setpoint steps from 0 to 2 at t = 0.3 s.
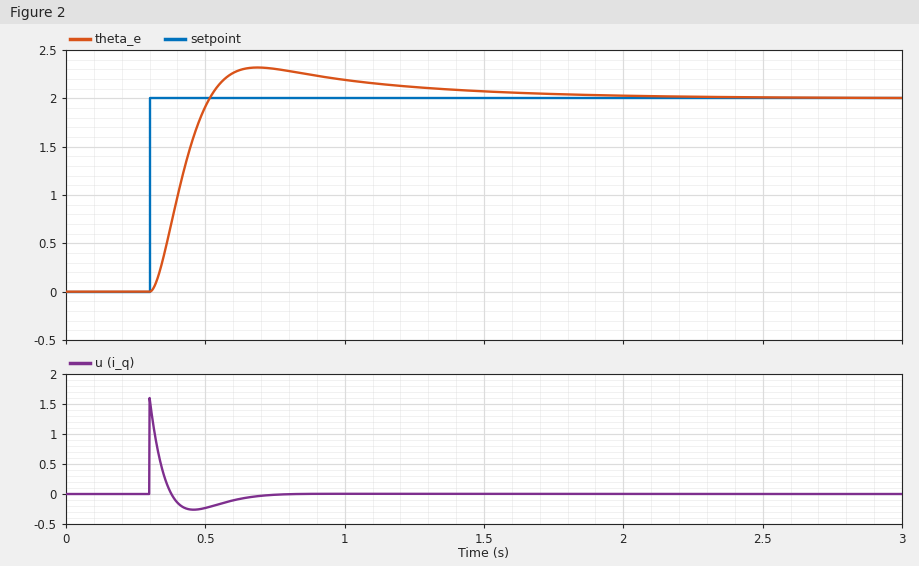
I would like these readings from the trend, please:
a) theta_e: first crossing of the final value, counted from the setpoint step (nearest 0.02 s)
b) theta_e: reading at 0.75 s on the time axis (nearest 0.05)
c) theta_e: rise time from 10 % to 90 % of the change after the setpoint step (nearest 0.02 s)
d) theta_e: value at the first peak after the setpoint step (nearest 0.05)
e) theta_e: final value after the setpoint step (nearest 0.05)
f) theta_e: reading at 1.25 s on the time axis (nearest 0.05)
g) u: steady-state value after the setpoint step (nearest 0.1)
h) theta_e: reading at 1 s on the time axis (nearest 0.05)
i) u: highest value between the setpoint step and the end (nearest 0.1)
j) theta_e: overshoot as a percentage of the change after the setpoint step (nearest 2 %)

0.22 s
2.30
0.14 s
2.30
2.00
2.10
0.0
2.20
1.6
16 %
